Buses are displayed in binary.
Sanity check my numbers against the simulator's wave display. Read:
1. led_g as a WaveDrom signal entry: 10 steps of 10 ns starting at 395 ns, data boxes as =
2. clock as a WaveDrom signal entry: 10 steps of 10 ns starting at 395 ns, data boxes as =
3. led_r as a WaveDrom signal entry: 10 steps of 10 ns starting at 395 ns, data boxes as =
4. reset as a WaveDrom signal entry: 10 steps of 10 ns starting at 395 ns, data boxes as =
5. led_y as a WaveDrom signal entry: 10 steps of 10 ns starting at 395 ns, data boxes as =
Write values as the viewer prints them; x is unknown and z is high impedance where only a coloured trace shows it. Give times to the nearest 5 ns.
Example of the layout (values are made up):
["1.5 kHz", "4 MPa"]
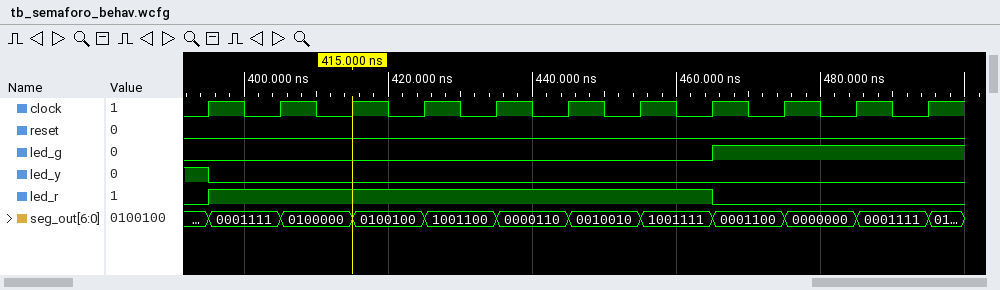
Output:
["{name: 'led_g', wave: '0......1..'}", "{name: 'clock', wave: 'p.........'}", "{name: 'led_r', wave: '1......0..'}", "{name: 'reset', wave: '0.........'}", "{name: 'led_y', wave: '0.........'}"]
